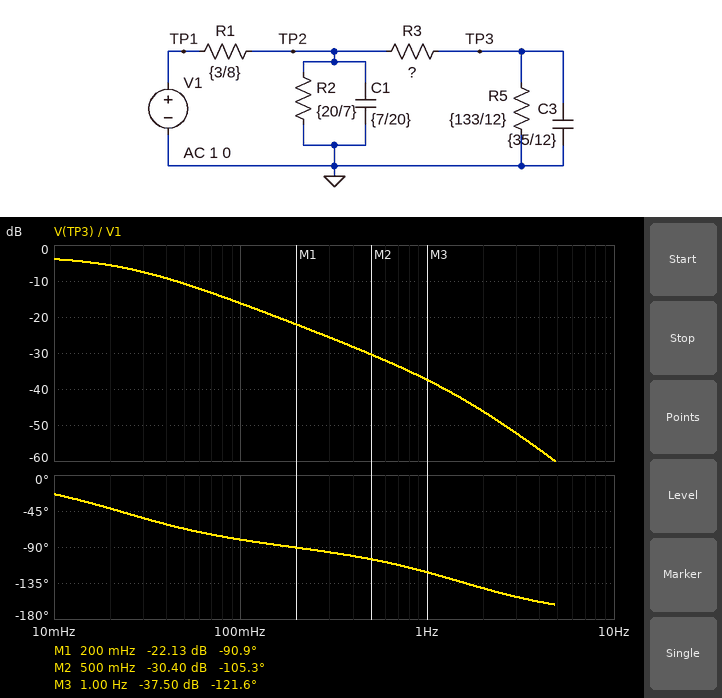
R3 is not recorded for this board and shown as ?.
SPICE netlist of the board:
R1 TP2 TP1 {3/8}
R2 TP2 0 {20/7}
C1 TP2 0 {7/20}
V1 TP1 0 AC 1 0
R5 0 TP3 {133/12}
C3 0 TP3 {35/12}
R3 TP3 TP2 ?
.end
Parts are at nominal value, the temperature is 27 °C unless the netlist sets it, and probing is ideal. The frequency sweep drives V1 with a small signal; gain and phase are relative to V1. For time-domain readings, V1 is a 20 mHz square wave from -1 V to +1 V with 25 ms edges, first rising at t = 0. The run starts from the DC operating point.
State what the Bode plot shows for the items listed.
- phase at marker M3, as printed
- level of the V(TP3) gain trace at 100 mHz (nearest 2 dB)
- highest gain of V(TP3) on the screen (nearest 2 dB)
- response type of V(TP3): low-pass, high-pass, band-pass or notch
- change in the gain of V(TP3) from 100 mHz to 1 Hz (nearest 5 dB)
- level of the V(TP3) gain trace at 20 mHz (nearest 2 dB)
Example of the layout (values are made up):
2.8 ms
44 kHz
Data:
-121.6 deg
-16 dB
-4 dB
low-pass
-20 dB
-6 dB
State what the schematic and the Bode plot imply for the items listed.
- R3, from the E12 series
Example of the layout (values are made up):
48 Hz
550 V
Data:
2.7 Ω
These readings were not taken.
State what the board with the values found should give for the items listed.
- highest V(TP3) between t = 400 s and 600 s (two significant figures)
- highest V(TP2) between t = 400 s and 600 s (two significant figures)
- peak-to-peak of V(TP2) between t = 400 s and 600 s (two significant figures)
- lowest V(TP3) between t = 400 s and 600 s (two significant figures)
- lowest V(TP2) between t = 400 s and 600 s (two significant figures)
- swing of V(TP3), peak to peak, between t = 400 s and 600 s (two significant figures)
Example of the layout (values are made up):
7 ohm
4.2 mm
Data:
660 mV
860 mV
1.7 V
-660 mV
-860 mV
1.3 V
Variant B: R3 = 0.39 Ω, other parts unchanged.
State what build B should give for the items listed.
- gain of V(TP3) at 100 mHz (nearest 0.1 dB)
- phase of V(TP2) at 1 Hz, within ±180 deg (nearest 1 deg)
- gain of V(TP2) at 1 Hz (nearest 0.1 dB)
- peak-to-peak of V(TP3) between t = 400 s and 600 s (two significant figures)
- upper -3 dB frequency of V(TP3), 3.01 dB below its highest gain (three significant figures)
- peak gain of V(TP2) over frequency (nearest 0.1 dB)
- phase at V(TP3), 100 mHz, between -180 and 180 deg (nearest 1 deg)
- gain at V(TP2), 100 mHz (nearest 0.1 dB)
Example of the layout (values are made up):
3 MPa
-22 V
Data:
-5.8 dB
-25 deg
-7.2 dB
1.7 V
78.4 mHz
-1.3 dB
-54 deg
-3.8 dB
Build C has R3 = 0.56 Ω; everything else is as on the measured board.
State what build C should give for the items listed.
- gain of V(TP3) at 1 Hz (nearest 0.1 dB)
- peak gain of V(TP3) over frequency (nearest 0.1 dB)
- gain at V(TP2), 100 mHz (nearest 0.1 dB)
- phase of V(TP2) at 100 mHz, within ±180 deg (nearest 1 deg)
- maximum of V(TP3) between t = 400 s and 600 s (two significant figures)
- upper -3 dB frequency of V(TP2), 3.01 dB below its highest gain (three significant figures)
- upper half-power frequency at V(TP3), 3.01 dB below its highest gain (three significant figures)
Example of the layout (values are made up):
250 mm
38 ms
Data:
-26.3 dB
-1.7 dB
-3.7 dB
-15 deg
820 mV
146 mHz
65.0 mHz
